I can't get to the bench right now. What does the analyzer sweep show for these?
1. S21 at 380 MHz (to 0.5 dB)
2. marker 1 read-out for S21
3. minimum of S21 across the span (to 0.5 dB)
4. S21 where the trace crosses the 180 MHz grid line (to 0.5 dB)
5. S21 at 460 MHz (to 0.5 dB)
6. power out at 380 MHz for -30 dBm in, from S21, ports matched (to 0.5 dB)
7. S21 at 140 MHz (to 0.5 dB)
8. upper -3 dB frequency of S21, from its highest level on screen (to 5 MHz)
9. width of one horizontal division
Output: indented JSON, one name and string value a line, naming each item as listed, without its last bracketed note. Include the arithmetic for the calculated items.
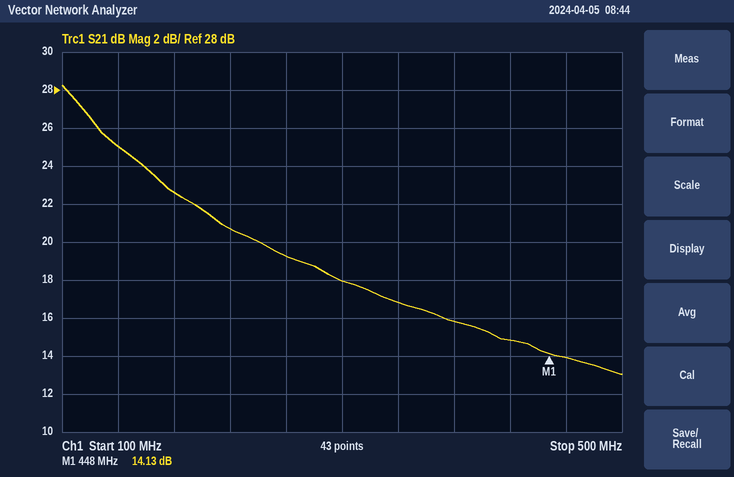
{
  "S21 at 380 MHz": "16.0 dB",
  "marker 1 read-out for S21": "14.13 dB",
  "minimum of S21 across the span": "13.0 dB",
  "S21 where the trace crosses the 180 MHz grid line": "22.5 dB",
  "S21 at 460 MHz": "14.0 dB",
  "power out at 380 MHz for -30 dBm in, from S21, ports matched": "-30 dBm + (16.0 dB) = -14.0 dBm",
  "S21 at 140 MHz": "25.0 dB",
  "upper -3 dB frequency of S21, from its highest level on screen": "135 MHz",
  "width of one horizontal division": "40 MHz"
}
